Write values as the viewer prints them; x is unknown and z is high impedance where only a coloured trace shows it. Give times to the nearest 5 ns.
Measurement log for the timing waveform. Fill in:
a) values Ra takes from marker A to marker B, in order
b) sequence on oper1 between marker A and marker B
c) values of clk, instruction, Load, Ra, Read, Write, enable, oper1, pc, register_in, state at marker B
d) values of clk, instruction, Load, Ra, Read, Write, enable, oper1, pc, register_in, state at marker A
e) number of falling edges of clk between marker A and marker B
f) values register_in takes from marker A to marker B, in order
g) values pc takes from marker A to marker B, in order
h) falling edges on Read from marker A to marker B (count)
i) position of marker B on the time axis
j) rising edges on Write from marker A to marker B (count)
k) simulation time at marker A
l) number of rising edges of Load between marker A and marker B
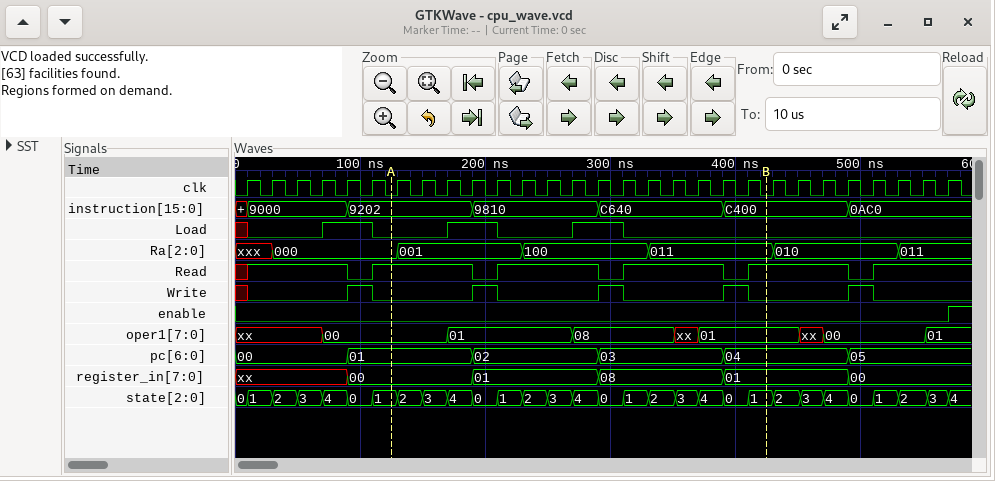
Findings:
000, 001, 100, 011
00, 01, 08, xx, 01
clk=0, instruction=C400, Load=0, Ra=011, Read=1, Write=0, enable=0, oper1=01, pc=04, register_in=01, state=1
clk=0, instruction=9202, Load=0, Ra=000, Read=1, Write=0, enable=0, oper1=00, pc=01, register_in=00, state=1
15
00, 01, 08, 01
01, 02, 03, 04
3
425 ns
3
125 ns
2
